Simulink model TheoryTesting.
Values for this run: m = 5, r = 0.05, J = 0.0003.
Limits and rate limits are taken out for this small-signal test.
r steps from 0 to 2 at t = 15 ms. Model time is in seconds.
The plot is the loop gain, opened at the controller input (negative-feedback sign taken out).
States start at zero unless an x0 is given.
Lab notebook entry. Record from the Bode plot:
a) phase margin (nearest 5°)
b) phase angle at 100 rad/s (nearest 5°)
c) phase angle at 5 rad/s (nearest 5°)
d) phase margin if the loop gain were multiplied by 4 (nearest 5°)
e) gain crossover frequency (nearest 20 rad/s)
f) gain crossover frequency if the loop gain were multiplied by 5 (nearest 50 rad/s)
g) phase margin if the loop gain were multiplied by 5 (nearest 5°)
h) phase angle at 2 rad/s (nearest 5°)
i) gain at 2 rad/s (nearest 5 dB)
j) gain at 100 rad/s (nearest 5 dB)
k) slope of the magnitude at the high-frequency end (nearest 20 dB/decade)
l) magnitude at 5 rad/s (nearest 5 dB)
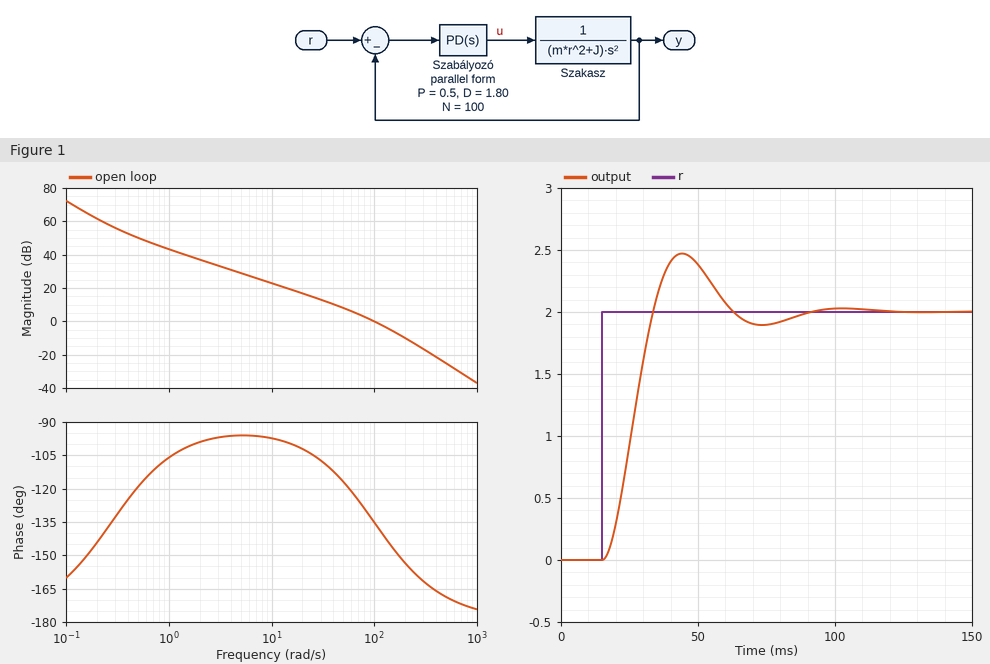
45°
-135°
-95°
25°
100 rad/s
250 rad/s
20°
-100°
35 dB
0 dB
-40 dB/decade
30 dB
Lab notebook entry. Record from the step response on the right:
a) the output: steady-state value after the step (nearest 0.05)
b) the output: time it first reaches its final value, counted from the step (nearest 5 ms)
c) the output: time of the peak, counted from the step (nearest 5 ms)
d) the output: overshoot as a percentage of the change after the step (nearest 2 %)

2.00
20 ms
30 ms
24 %
